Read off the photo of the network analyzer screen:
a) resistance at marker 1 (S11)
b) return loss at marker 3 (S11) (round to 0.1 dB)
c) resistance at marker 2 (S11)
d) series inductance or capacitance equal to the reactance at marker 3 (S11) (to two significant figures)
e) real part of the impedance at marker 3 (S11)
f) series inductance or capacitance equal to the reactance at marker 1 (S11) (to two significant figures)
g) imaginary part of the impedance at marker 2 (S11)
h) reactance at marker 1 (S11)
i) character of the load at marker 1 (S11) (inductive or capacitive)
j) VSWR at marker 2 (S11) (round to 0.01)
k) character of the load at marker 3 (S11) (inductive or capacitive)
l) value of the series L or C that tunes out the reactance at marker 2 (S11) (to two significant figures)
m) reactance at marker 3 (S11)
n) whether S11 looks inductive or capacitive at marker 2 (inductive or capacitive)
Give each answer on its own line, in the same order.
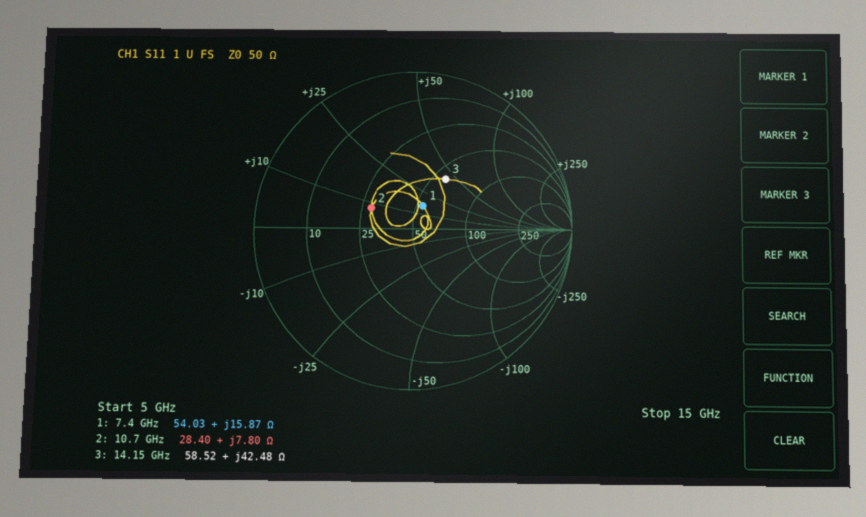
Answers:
54.03 Ω
8.6 dB
28.40 Ω
480 pH
58.52 Ω
340 pH
+7.80 Ω
+15.87 Ω
inductive
1.82
inductive
1.9 pF
+42.48 Ω
inductive
